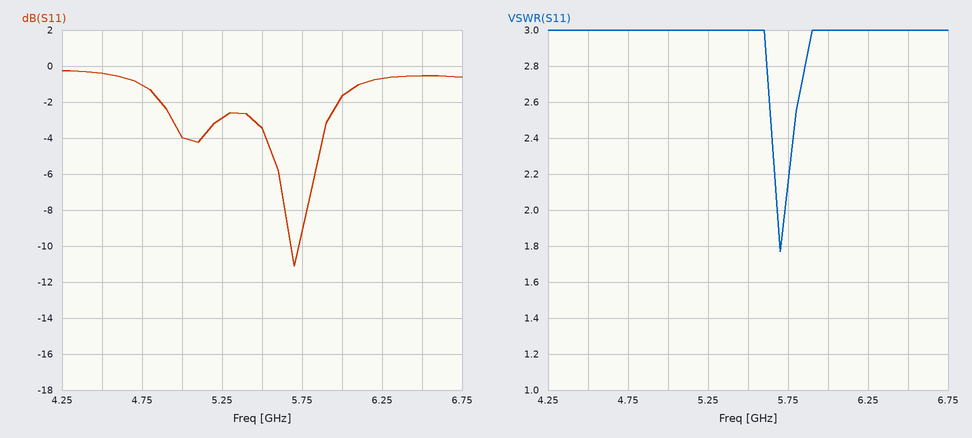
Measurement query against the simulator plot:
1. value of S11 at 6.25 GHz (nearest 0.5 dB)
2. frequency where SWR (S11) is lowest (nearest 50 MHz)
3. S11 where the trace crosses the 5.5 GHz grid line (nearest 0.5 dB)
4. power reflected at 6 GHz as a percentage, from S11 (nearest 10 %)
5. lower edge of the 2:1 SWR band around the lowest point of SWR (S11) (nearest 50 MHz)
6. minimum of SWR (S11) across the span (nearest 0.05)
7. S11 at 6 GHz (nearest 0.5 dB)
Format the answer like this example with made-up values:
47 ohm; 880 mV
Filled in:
-0.5 dB; 5.70 GHz; -3.5 dB; 70 %; 5.70 GHz; 1.75; -1.5 dB
